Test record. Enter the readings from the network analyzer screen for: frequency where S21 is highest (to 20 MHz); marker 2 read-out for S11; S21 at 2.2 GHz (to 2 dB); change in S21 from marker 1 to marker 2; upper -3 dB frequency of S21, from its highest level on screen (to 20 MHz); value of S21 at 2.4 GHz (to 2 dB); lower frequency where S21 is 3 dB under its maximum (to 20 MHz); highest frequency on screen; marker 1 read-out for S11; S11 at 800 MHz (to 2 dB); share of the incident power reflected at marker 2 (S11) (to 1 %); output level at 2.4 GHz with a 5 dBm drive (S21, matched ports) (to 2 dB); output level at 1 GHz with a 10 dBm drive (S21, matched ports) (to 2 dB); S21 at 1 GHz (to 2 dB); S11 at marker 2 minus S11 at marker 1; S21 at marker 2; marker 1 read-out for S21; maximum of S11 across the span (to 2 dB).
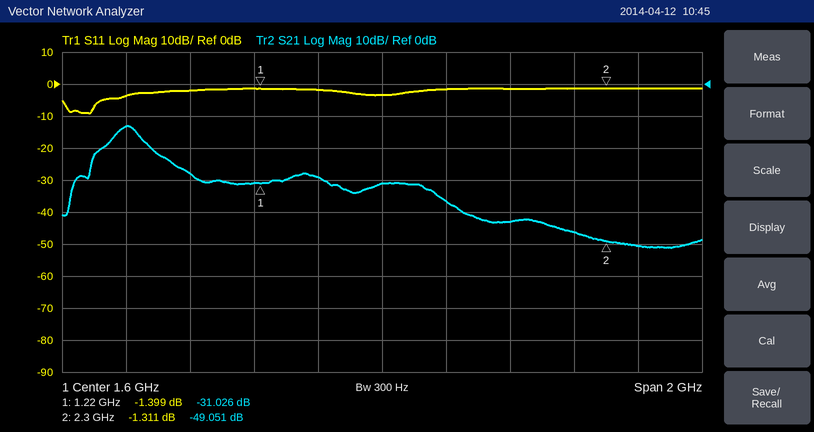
800 MHz
-1.311 dB
-46 dB
-18.025 dB
840 MHz
-50 dB
760 MHz
2.6 GHz
-1.399 dB
-4 dB
74 %
-46 dBm
-18 dBm
-28 dB
0.088 dB
-49.051 dB
-31.026 dB
-2 dB
